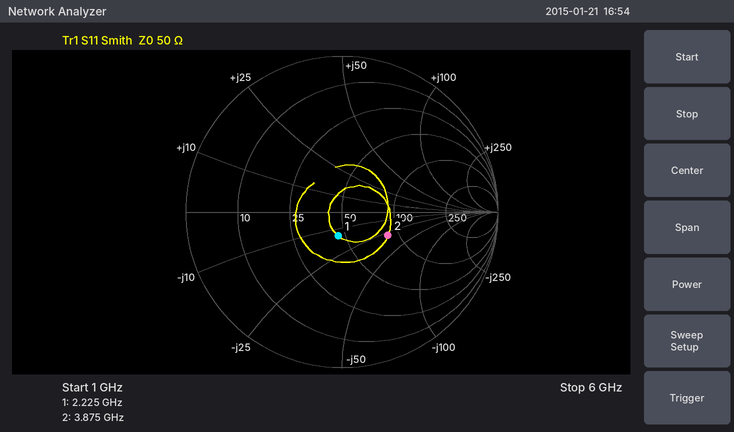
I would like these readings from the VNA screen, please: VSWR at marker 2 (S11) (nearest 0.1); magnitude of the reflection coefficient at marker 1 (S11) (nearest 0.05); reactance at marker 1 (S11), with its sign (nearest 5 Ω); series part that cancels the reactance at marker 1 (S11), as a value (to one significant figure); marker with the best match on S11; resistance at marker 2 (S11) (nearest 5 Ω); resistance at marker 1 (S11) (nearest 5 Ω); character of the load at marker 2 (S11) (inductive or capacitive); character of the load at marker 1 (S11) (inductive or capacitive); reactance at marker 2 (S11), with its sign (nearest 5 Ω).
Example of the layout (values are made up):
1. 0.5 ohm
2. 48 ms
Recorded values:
1. 2.0
2. 0.15
3. -15 Ω
4. 1 nH
5. marker 1
6. 85 Ω
7. 45 Ω
8. capacitive
9. capacitive
10. -30 Ω
